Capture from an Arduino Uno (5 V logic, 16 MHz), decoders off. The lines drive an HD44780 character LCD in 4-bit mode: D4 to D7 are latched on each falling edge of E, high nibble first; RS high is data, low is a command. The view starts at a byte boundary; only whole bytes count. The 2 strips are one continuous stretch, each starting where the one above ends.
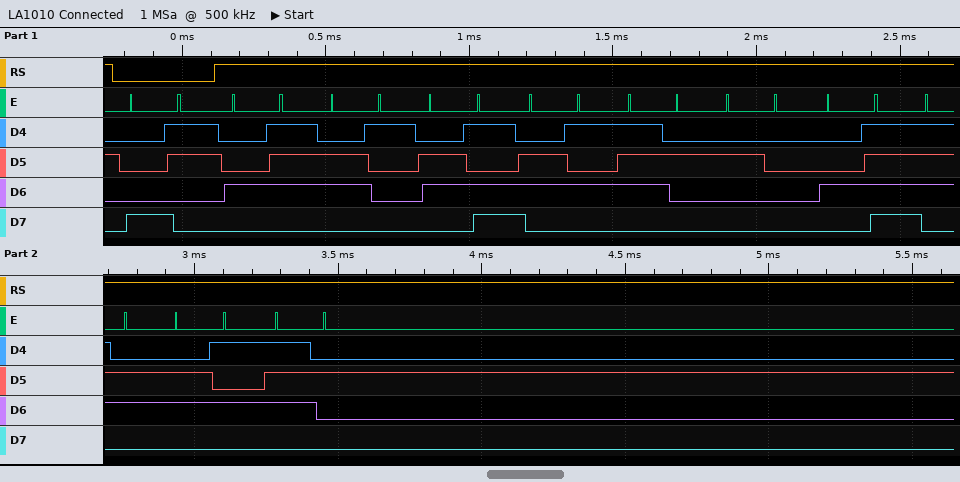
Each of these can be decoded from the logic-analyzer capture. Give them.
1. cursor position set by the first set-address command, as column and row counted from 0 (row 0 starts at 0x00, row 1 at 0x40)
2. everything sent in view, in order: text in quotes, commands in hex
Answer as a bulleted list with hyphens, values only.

- column 3, row 0
- 0x83 "Gamer Over"
